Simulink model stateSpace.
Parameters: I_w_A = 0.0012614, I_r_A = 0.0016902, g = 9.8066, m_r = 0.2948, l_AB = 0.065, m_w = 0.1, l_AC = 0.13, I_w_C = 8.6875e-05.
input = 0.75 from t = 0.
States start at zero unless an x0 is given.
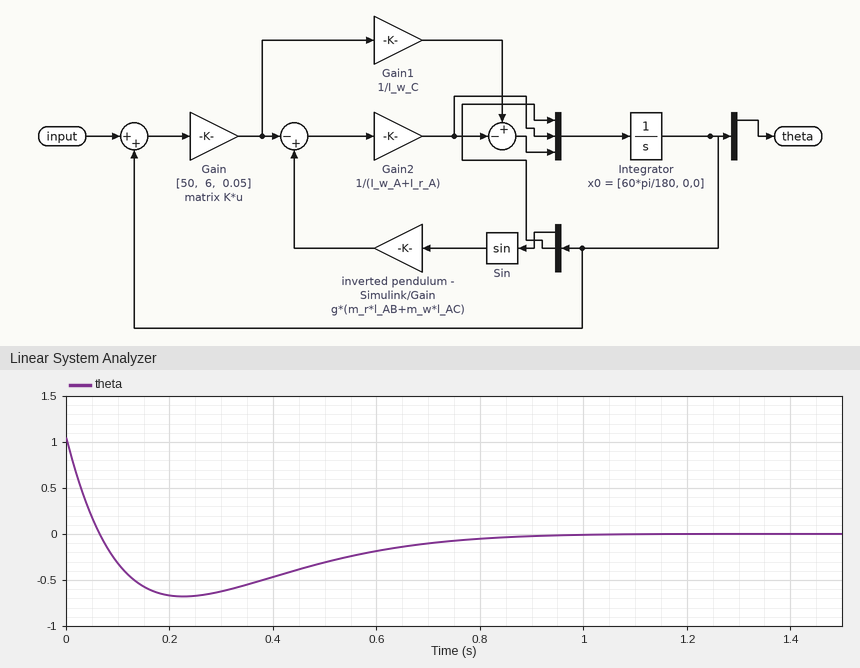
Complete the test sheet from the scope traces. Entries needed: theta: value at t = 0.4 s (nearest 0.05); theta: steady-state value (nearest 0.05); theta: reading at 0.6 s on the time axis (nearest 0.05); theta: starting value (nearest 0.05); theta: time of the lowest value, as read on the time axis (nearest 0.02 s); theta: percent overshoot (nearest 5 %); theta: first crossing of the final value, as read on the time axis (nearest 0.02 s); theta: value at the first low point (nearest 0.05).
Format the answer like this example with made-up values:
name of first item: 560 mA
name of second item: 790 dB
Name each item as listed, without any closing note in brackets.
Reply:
theta: value at t = 0.4 s: -0.45
theta: steady-state value: 0.00
theta: reading at 0.6 s on the time axis: -0.20
theta: starting value: 1.05
theta: time of the lowest value, as read on the time axis: 0.22 s
theta: percent overshoot: 65 %
theta: first crossing of the final value, as read on the time axis: 0.06 s
theta: value at the first low point: -0.70
